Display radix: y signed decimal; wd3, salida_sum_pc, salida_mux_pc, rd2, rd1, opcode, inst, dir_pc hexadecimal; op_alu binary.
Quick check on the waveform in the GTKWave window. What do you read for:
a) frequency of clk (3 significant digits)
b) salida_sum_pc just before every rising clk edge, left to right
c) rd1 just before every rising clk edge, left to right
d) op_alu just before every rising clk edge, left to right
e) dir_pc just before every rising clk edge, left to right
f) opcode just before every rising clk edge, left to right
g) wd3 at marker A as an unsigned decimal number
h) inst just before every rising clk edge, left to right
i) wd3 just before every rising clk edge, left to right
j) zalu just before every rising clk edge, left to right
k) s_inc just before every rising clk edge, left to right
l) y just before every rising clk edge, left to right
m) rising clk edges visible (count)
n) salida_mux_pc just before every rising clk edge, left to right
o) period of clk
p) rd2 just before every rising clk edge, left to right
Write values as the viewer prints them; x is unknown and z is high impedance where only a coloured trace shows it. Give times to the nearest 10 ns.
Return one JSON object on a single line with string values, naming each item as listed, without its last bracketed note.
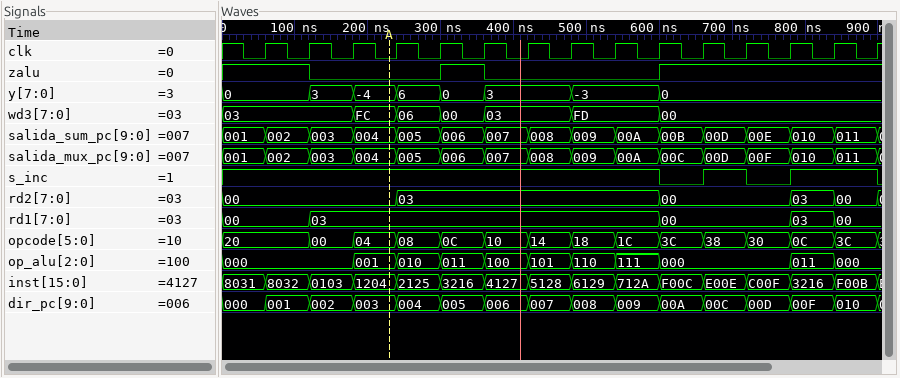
{"frequency of clk": "16.7 MHz", "salida_sum_pc just before every rising clk edge, left to right": "001, 002, 003, 004, 005, 006, 007, 008, 009, 00A, 00B, 00D, 00E, 010, 011", "rd1 just before every rising clk edge, left to right": "00, 00, 03, 03, 03, 03, 03, 03, 03, 03, 00, 00, 00, 03, 00", "op_alu just before every rising clk edge, left to right": "000, 000, 000, 001, 010, 011, 100, 101, 110, 111, 000, 000, 000, 011, 000", "dir_pc just before every rising clk edge, left to right": "000, 001, 002, 003, 004, 005, 006, 007, 008, 009, 00A, 00C, 00D, 00F, 010", "opcode just before every rising clk edge, left to right": "20, 20, 00, 04, 08, 0C, 10, 14, 18, 1C, 3C, 38, 30, 0C, 3C", "wd3 at marker A as an unsigned decimal number": "252", "inst just before every rising clk edge, left to right": "8031, 8032, 0103, 1204, 2125, 3216, 4127, 5128, 6129, 712A, F00C, E00E, C00F, 3216, F00B", "wd3 just before every rising clk edge, left to right": "03, 03, 03, FC, 06, 00, 03, 03, FD, FD, 00, 00, 00, 00, 00", "zalu just before every rising clk edge, left to right": "1 1 0 0 0 1 0 0 0 0 1 1 1 1 1", "s_inc just before every rising clk edge, left to right": "1 1 1 1 1 1 1 1 1 1 0 1 0 1 1", "y just before every rising clk edge, left to right": "0, 0, 3, -4, 6, 0, 3, 3, -3, -3, 0, 0, 0, 0, 0", "rising clk edges visible": "15", "salida_mux_pc just before every rising clk edge, left to right": "001, 002, 003, 004, 005, 006, 007, 008, 009, 00A, 00C, 00D, 00F, 010, 011", "period of clk": "60 ns", "rd2 just before every rising clk edge, left to right": "00, 00, 00, 00, 03, 03, 03, 03, 03, 03, 00, 00, 00, 03, 00"}
